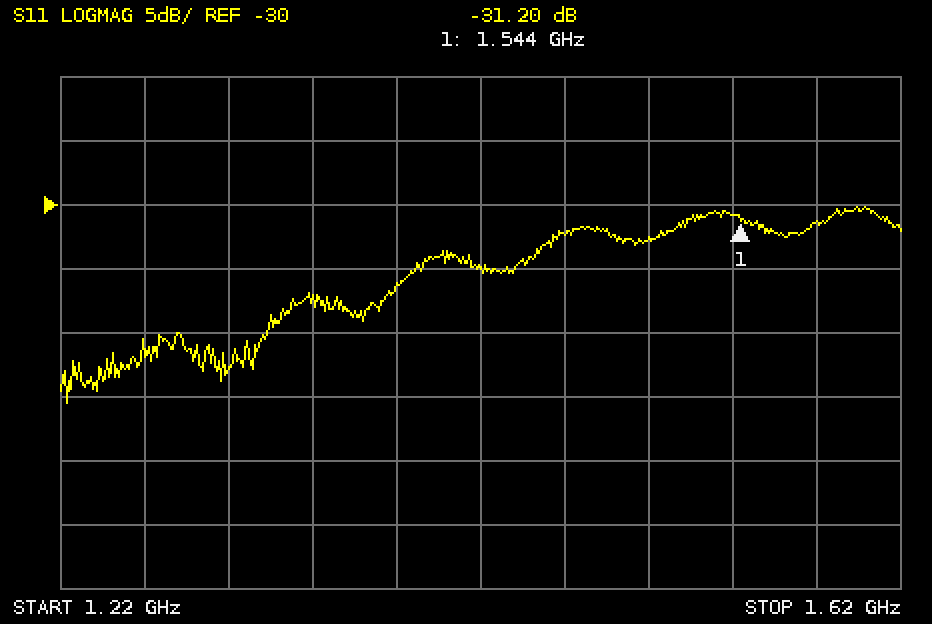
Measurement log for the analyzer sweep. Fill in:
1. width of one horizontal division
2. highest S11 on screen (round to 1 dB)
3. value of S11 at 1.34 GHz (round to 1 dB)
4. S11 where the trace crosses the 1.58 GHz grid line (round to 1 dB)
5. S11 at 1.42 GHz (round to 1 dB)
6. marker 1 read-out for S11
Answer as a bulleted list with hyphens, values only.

- 40 MHz
- -30 dB
- -37 dB
- -31 dB
- -35 dB
- -31.20 dB
